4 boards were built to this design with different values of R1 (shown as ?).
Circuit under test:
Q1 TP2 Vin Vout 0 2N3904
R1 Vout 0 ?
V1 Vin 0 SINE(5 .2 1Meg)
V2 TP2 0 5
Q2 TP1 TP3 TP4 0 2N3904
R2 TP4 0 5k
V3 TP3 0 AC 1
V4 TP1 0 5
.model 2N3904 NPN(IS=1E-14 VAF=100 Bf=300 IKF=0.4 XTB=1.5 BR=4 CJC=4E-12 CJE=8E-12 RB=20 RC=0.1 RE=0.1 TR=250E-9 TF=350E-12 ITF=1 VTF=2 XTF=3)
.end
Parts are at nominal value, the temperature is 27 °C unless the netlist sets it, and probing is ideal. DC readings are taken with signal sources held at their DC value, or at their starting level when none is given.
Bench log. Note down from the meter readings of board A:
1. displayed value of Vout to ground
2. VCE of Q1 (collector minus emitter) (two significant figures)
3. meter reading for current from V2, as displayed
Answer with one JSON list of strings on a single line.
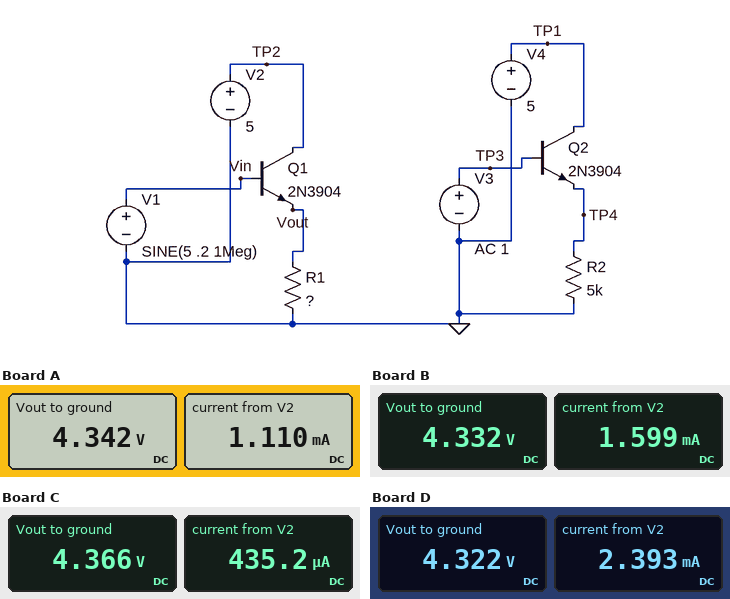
["4.342 V", "660 mV", "1.110 mA"]
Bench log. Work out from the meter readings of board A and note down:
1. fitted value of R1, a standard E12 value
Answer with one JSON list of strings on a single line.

["3.9 kΩ"]
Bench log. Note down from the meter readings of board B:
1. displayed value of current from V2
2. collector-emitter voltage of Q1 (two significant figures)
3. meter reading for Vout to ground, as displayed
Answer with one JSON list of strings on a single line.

["1.599 mA", "670 mV", "4.332 V"]
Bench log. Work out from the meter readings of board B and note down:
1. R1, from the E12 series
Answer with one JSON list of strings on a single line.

["2.7 kΩ"]
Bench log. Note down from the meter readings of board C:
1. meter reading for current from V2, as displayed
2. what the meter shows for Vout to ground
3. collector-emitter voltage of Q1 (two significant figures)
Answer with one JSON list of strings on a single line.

["435.2 µA", "4.366 V", "630 mV"]
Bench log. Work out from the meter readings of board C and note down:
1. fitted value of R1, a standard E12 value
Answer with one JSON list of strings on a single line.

["10 kΩ"]
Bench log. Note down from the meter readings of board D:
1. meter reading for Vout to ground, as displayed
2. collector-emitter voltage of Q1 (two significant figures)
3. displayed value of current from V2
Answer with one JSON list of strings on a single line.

["4.322 V", "680 mV", "2.393 mA"]
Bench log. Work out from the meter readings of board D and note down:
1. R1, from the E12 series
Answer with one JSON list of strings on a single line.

["1.8 kΩ"]
